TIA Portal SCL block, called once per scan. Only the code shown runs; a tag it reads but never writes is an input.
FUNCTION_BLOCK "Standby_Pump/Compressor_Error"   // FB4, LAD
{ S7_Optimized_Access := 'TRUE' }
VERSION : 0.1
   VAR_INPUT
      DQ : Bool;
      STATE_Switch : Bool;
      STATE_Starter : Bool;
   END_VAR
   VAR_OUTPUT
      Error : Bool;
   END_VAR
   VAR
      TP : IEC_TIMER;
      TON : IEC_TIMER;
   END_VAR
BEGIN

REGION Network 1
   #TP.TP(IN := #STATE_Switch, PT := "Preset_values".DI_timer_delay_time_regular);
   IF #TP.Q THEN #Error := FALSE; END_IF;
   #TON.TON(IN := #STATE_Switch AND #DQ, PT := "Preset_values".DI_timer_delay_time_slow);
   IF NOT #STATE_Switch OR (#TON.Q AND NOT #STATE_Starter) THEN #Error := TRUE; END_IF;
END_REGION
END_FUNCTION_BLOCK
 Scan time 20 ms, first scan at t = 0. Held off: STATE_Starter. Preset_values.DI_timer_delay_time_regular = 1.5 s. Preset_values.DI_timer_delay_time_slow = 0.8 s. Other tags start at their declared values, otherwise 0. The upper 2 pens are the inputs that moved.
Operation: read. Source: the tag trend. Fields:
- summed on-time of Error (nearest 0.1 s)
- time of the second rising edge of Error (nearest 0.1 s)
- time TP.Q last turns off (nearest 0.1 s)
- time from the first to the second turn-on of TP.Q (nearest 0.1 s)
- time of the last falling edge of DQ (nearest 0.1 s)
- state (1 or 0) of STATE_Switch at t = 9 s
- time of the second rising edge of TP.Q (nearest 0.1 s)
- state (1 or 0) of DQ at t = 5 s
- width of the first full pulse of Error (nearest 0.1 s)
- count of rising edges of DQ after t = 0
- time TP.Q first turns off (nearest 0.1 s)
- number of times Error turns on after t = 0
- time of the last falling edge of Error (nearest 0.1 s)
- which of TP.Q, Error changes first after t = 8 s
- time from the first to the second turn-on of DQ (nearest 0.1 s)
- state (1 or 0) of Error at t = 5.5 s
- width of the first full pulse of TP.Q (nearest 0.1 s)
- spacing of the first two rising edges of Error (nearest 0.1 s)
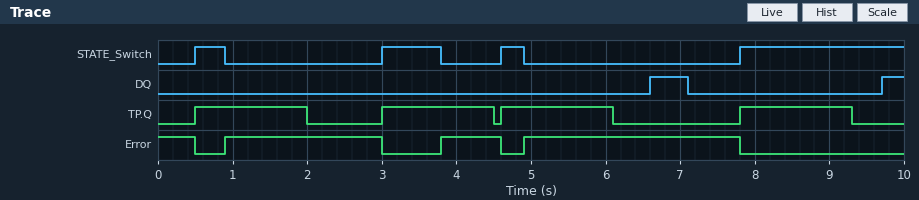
6.3 s
3.8 s
9.3 s
2.5 s
7.1 s
1
3.0 s
0
2.1 s
2
2.0 s
3
7.8 s
TP.Q
3.1 s
1
1.5 s
2.9 s
